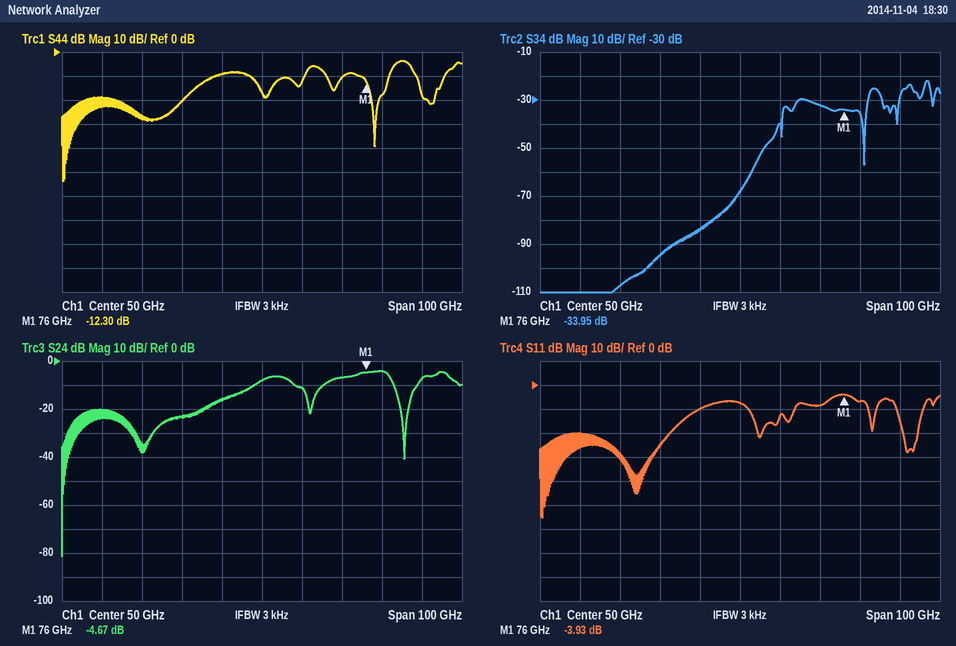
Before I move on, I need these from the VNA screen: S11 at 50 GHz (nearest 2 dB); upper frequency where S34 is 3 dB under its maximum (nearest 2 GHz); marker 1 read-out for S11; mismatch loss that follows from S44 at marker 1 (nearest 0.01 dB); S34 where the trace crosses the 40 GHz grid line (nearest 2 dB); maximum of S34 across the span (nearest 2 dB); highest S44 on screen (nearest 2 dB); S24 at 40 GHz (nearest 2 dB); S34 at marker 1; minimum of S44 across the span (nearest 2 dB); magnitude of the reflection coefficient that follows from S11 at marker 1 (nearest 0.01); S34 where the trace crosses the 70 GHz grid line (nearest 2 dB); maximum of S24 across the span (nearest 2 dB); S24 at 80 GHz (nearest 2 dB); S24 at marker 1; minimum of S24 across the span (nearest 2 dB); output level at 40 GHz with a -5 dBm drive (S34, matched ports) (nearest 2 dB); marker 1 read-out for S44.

-8 dB
98 GHz
-3.93 dB
0.26 dB
-84 dB
-22 dB
-4 dB
-16 dB
-33.95 dB
-54 dB
0.64
-32 dB
-4 dB
-4 dB
-4.67 dB
-82 dB
-88 dBm
-12.30 dB
